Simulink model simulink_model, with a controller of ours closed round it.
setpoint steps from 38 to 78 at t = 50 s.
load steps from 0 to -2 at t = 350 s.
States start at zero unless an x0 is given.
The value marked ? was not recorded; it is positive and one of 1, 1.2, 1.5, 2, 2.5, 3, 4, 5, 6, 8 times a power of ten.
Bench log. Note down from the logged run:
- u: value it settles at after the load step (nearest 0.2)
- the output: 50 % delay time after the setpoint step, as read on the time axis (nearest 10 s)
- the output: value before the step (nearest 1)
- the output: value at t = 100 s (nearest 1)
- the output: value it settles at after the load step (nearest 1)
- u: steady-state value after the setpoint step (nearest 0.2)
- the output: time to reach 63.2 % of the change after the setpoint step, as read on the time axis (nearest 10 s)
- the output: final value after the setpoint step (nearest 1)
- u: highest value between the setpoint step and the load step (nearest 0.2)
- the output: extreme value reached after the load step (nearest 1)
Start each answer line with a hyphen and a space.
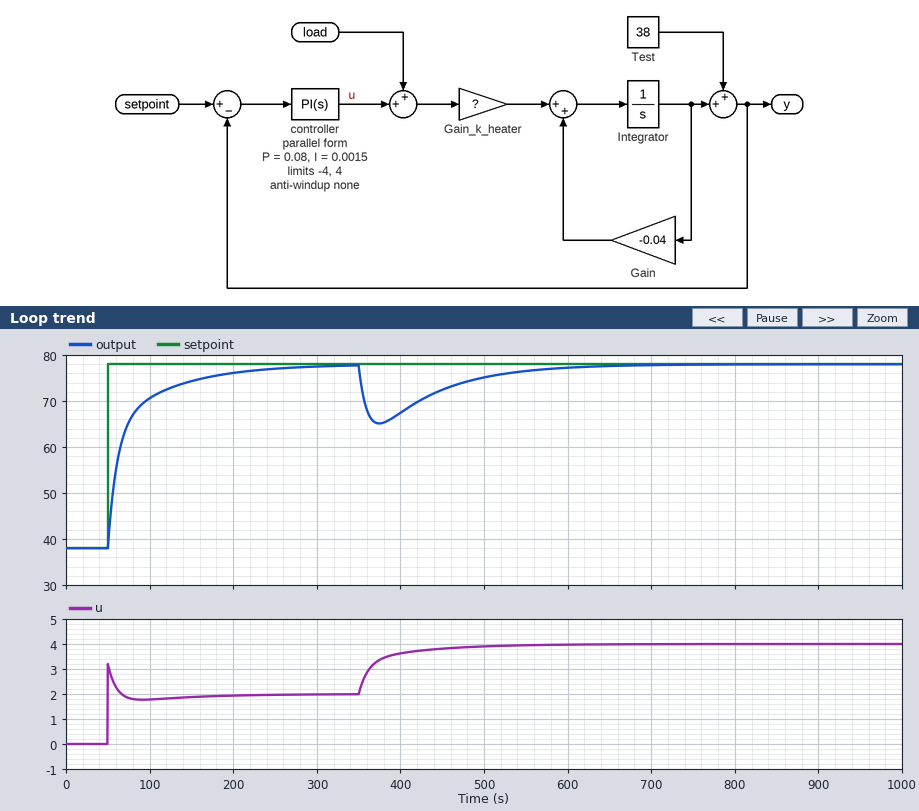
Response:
- 4.0
- 60 s
- 38
- 71
- 78
- 2.0
- 70 s
- 78
- 3.2
- 65
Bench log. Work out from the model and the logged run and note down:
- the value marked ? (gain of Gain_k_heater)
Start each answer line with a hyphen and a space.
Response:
- 0.8
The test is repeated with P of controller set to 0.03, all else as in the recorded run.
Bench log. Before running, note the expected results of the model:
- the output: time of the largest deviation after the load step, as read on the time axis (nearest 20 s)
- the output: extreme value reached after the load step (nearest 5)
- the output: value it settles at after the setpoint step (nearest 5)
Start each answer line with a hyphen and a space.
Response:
- 380 s
- 60
- 80
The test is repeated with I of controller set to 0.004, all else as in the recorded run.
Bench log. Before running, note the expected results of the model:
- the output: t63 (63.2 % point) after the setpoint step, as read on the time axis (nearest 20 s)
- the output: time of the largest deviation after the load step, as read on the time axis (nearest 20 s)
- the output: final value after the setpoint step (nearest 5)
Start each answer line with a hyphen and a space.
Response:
- 60 s
- 360 s
- 80
